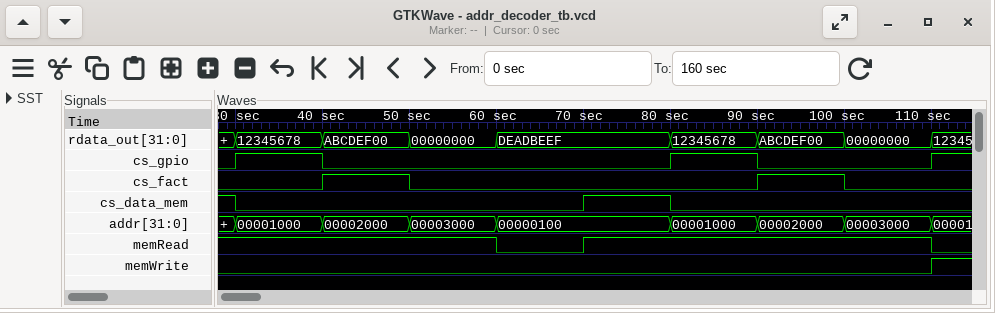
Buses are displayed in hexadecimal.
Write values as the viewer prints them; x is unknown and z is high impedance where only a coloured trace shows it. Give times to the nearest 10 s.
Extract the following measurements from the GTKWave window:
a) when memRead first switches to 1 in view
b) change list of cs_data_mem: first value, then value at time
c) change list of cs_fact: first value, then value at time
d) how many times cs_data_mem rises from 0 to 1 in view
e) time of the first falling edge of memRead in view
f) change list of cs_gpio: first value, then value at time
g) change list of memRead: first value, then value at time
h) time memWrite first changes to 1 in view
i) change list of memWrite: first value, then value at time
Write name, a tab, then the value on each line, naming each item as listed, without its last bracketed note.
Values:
when memRead first switches to 1 in view	70 s
change list of cs_data_mem: first value, then value at time	1, 0 at 30 s, 1 at 70 s, 0 at 80 s
change list of cs_fact: first value, then value at time	0, 1 at 40 s, 0 at 50 s, 1 at 90 s, 0 at 100 s
how many times cs_data_mem rises from 0 to 1 in view	1
time of the first falling edge of memRead in view	60 s
change list of cs_gpio: first value, then value at time	0, 1 at 30 s, 0 at 40 s, 1 at 80 s, 0 at 90 s, 1 at 110 s
change list of memRead: first value, then value at time	1, 0 at 60 s, 1 at 70 s, 0 at 110 s
time memWrite first changes to 1 in view	110 s
change list of memWrite: first value, then value at time	0, 1 at 110 s
